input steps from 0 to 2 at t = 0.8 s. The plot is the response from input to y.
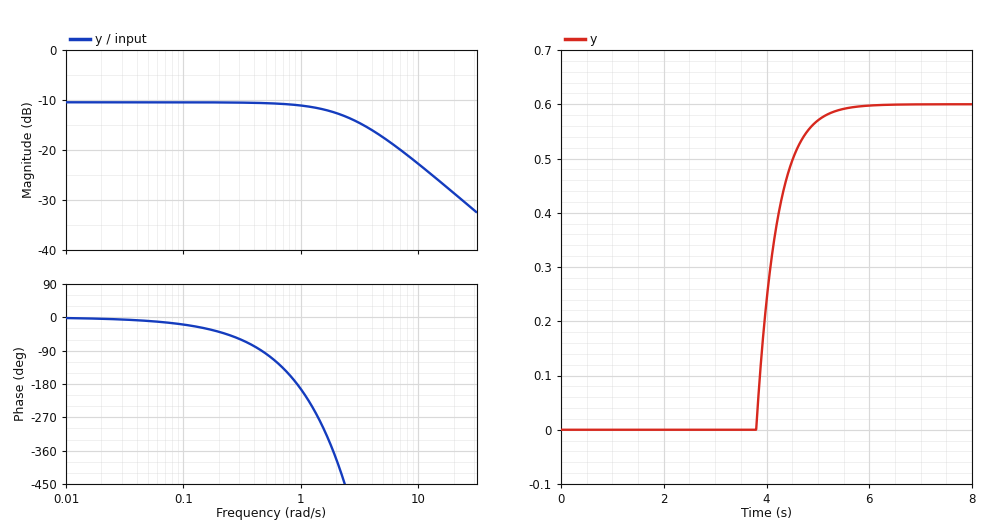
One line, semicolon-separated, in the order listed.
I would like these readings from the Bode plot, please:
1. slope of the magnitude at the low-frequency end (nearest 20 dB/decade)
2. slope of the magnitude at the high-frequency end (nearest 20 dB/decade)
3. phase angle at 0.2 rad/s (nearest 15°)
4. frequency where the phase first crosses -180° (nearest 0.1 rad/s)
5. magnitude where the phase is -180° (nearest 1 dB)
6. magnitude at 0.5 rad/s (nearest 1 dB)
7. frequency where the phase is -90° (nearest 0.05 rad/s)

0 dB/decade; -20 dB/decade; -45°; 0.9 rad/s; -11 dB; -11 dB; 0.45 rad/s
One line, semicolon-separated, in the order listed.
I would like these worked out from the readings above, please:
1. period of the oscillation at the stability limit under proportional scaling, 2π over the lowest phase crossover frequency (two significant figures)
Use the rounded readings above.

7.0 s
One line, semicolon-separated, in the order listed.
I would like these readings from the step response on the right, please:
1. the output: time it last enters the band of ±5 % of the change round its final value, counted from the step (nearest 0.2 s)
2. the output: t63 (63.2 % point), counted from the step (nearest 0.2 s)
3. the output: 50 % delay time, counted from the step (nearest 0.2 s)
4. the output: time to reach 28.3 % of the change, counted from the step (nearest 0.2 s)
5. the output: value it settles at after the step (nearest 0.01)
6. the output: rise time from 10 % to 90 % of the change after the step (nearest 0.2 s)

4.2 s; 3.4 s; 3.2 s; 3.2 s; 0.60; 0.8 s
